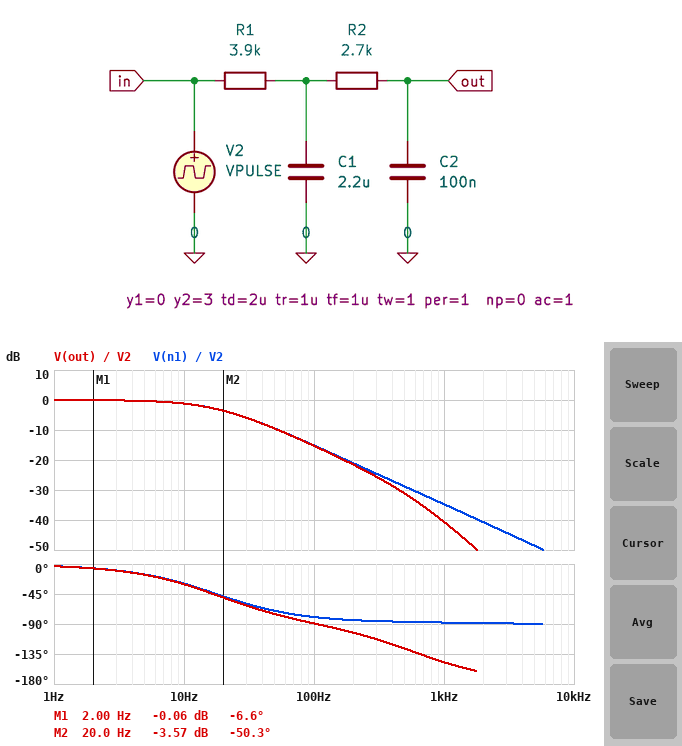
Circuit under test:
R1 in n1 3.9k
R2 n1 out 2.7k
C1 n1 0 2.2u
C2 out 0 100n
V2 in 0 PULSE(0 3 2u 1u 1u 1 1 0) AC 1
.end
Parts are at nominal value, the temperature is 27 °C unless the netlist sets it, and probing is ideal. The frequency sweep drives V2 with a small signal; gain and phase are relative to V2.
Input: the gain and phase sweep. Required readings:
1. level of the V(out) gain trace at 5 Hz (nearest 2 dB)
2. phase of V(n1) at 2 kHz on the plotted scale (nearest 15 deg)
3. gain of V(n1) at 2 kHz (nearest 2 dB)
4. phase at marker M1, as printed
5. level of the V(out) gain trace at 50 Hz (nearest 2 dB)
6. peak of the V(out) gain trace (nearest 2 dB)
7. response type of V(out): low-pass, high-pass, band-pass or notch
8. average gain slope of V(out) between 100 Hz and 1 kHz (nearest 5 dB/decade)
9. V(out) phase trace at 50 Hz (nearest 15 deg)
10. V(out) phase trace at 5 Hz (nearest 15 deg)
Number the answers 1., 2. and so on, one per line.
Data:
1. 0 dB
2. -90 deg
3. -40 dB
4. -6.6 deg
5. -10 dB
6. 0 dB
7. low-pass
8. -25 dB/decade
9. -75 deg
10. -15 deg
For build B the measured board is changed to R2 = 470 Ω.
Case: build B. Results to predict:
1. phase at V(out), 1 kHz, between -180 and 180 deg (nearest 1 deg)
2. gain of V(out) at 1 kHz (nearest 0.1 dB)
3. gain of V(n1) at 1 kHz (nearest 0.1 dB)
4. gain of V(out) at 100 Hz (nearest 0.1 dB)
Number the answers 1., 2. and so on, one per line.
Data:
1. -105 deg
2. -35.4 dB
3. -35.0 dB
4. -15.2 dB
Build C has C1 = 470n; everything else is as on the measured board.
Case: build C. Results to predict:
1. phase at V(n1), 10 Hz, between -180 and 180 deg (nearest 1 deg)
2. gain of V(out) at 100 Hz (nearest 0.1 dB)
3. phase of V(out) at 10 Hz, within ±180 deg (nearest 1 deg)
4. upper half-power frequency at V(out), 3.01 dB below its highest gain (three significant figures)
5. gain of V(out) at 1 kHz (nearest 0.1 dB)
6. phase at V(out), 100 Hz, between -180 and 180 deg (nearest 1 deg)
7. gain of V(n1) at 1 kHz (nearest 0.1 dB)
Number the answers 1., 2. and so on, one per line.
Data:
1. -8 deg
2. -4.9 dB
3. -9 deg
4. 69.3 Hz
5. -27.7 dB
6. -63 deg
7. -21.8 dB
